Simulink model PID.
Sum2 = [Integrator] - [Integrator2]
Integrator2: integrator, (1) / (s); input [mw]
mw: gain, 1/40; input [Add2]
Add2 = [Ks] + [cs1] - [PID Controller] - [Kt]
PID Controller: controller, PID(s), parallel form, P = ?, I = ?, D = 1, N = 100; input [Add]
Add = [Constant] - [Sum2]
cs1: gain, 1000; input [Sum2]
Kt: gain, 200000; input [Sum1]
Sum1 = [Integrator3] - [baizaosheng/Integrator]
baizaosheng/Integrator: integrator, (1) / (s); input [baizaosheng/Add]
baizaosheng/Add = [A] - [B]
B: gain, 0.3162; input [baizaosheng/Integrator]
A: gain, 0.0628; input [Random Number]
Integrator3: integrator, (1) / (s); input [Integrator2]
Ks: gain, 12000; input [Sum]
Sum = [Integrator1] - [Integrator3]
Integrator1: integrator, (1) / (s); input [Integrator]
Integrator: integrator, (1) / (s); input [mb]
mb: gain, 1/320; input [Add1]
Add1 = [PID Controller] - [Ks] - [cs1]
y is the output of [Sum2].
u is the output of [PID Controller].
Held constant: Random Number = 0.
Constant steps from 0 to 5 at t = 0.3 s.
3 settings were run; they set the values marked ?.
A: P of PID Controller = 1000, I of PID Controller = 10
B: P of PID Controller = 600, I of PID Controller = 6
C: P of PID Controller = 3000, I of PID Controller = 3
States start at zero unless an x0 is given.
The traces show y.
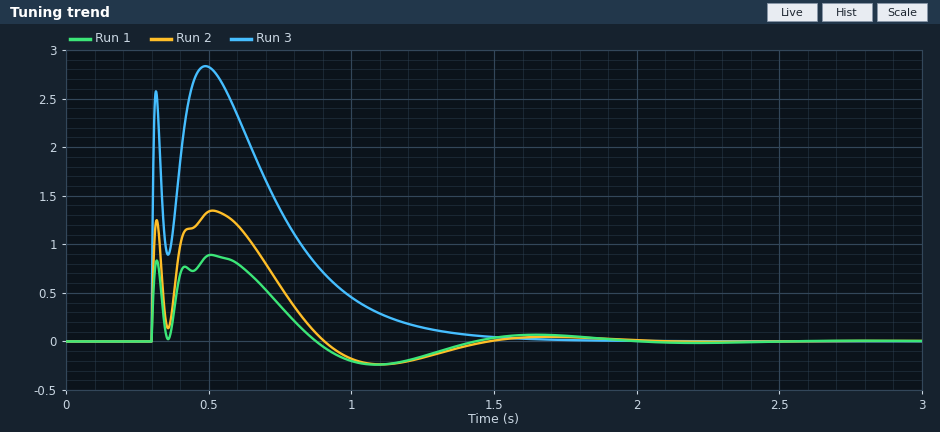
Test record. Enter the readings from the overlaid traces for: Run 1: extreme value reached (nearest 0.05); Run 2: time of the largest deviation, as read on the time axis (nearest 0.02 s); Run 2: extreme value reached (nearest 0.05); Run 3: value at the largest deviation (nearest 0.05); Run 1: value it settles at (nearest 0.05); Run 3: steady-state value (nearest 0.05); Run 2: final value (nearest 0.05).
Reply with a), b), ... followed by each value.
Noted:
a) 0.90
b) 0.52 s
c) 1.35
d) 2.85
e) 0.00
f) 0.00
g) 0.00
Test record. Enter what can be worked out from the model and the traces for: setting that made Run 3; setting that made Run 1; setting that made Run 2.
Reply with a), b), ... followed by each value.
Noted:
a) C
b) B
c) A
